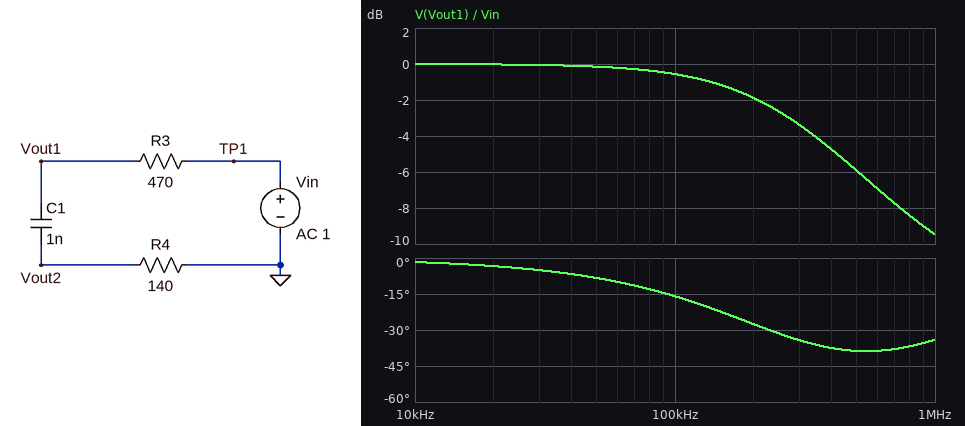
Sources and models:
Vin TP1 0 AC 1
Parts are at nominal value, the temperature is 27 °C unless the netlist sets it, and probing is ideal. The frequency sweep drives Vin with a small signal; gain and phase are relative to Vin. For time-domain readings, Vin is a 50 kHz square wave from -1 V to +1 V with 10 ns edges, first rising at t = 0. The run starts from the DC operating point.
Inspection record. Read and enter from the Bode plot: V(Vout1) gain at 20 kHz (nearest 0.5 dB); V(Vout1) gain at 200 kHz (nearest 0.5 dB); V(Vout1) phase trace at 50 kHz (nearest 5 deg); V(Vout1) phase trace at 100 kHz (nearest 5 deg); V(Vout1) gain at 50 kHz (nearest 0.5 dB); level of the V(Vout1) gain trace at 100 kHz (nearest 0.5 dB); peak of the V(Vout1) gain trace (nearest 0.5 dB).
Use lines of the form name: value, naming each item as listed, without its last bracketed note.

V(Vout1) gain at 20 kHz: 0 dB
V(Vout1) gain at 200 kHz: -2.0 dB
V(Vout1) phase trace at 50 kHz: -10 deg
V(Vout1) phase trace at 100 kHz: -15 deg
V(Vout1) gain at 50 kHz: 0 dB
level of the V(Vout1) gain trace at 100 kHz: -0.5 dB
peak of the V(Vout1) gain trace: 0 dB
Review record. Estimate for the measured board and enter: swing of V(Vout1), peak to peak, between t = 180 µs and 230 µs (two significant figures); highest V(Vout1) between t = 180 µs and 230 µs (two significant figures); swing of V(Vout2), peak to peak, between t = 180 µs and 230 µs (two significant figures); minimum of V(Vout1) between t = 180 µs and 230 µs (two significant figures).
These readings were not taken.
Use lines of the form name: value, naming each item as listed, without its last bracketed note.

swing of V(Vout1), peak to peak, between t = 180 µs and 230 µs: 2.0 V
highest V(Vout1) between t = 180 µs and 230 µs: 1.0 V
swing of V(Vout2), peak to peak, between t = 180 µs and 230 µs: 910 mV
minimum of V(Vout1) between t = 180 µs and 230 µs: -1.0 V
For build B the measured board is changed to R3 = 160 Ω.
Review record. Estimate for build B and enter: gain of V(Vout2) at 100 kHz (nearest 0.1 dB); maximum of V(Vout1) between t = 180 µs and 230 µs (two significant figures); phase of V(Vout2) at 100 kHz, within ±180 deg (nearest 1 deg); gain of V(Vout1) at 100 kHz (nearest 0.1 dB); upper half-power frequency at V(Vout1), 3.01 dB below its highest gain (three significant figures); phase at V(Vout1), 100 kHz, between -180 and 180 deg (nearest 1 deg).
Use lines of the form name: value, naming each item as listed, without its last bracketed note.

gain of V(Vout2) at 100 kHz: -21.3 dB
maximum of V(Vout1) between t = 180 µs and 230 µs: 1.0 V
phase of V(Vout2) at 100 kHz, within ±180 deg: 79 deg
gain of V(Vout1) at 100 kHz: -0.1 dB
upper half-power frequency at V(Vout1), 3.01 dB below its highest gain: 706 kHz
phase at V(Vout1), 100 kHz, between -180 and 180 deg: -6 deg
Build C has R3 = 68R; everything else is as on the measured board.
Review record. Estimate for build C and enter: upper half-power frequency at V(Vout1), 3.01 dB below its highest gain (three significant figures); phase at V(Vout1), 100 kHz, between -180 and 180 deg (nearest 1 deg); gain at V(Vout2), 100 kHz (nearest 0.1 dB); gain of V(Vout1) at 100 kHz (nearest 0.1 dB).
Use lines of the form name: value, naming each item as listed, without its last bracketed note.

upper half-power frequency at V(Vout1), 3.01 dB below its highest gain: 2.50 MHz
phase at V(Vout1), 100 kHz, between -180 and 180 deg: -2 deg
gain at V(Vout2), 100 kHz: -21.2 dB
gain of V(Vout1) at 100 kHz: 0 dB
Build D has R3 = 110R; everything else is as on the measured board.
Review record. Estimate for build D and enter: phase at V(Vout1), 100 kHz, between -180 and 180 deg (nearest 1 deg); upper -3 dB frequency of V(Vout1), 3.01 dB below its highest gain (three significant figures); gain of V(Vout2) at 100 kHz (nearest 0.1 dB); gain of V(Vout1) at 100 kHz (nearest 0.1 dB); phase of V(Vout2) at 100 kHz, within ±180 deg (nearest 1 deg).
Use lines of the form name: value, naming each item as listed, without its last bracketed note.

phase at V(Vout1), 100 kHz, between -180 and 180 deg: -4 deg
upper -3 dB frequency of V(Vout1), 3.01 dB below its highest gain: 1.04 MHz
gain of V(Vout2) at 100 kHz: -21.2 dB
gain of V(Vout1) at 100 kHz: -0.1 dB
phase of V(Vout2) at 100 kHz, within ±180 deg: 81 deg
